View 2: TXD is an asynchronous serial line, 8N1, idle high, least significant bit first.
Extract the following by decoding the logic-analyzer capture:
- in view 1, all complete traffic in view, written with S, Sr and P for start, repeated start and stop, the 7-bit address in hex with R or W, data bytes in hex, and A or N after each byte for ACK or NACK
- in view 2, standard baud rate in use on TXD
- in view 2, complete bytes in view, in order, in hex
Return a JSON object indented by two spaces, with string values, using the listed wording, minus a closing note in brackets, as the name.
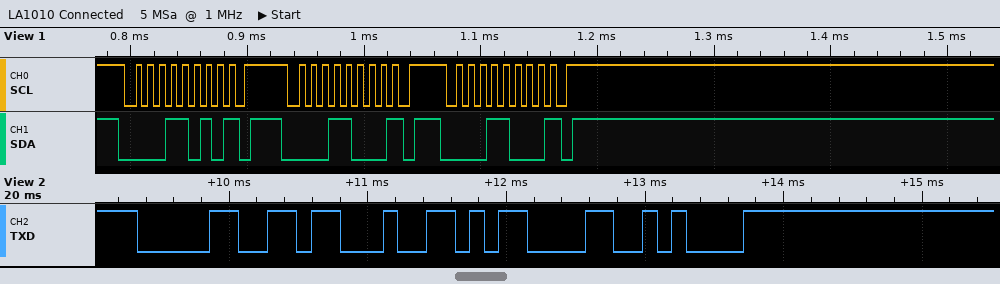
{
  "in view 1, all complete traffic in view, written with S, Sr and P for start, repeated start and stop, the 7-bit address in hex with R or W, data bytes in hex, and A or N after each byte for ACK or NACK": "S 0DW N P S 0CW N P S 0CW N P",
  "in view 2, standard baud rate in use on TXD": "9600 baud",
  "in view 2, complete bytes in view, in order, in hex": "30 23 0D 0A"
}
